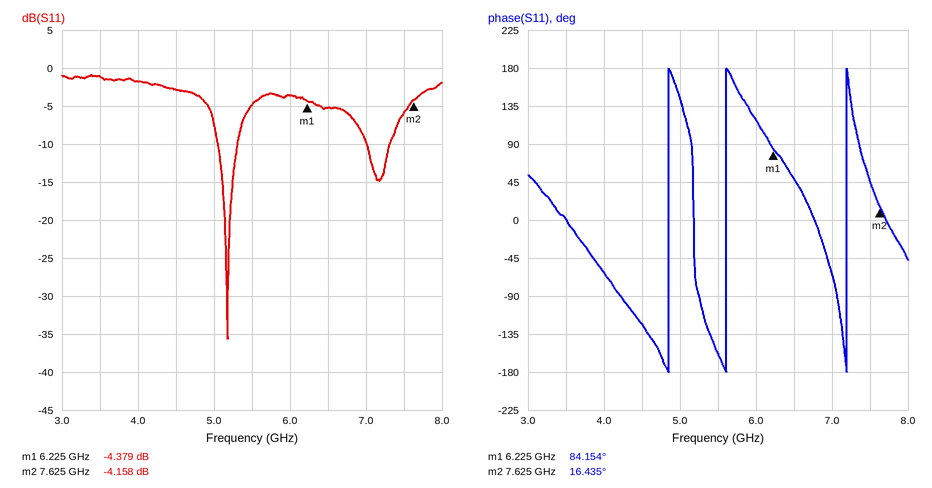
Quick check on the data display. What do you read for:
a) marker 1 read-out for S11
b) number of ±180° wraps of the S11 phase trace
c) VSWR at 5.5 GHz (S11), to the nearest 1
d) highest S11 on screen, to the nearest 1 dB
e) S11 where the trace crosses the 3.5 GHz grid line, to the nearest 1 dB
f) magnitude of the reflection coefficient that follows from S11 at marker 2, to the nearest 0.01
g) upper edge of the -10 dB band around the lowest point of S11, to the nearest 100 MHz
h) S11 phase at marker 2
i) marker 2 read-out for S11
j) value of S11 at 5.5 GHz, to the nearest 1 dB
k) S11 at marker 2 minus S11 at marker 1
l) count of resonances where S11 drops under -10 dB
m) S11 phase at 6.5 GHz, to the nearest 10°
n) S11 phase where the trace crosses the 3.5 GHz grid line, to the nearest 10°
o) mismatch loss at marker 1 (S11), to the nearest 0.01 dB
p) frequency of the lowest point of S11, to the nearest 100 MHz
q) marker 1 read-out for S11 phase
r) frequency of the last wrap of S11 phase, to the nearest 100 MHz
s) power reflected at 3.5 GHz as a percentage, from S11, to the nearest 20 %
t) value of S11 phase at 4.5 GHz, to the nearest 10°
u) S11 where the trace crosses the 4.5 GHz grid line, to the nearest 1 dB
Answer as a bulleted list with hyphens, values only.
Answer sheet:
- -4.379 dB
- 3
- 4
- -1 dB
- -1 dB
- 0.62
- 5.3 GHz
- 16.435°
- -4.158 dB
- -5 dB
- 0.221 dB
- 2
- 50°
- 0°
- 1.97 dB
- 5.2 GHz
- 84.154°
- 7.2 GHz
- 80 %
- -120°
- -3 dB
